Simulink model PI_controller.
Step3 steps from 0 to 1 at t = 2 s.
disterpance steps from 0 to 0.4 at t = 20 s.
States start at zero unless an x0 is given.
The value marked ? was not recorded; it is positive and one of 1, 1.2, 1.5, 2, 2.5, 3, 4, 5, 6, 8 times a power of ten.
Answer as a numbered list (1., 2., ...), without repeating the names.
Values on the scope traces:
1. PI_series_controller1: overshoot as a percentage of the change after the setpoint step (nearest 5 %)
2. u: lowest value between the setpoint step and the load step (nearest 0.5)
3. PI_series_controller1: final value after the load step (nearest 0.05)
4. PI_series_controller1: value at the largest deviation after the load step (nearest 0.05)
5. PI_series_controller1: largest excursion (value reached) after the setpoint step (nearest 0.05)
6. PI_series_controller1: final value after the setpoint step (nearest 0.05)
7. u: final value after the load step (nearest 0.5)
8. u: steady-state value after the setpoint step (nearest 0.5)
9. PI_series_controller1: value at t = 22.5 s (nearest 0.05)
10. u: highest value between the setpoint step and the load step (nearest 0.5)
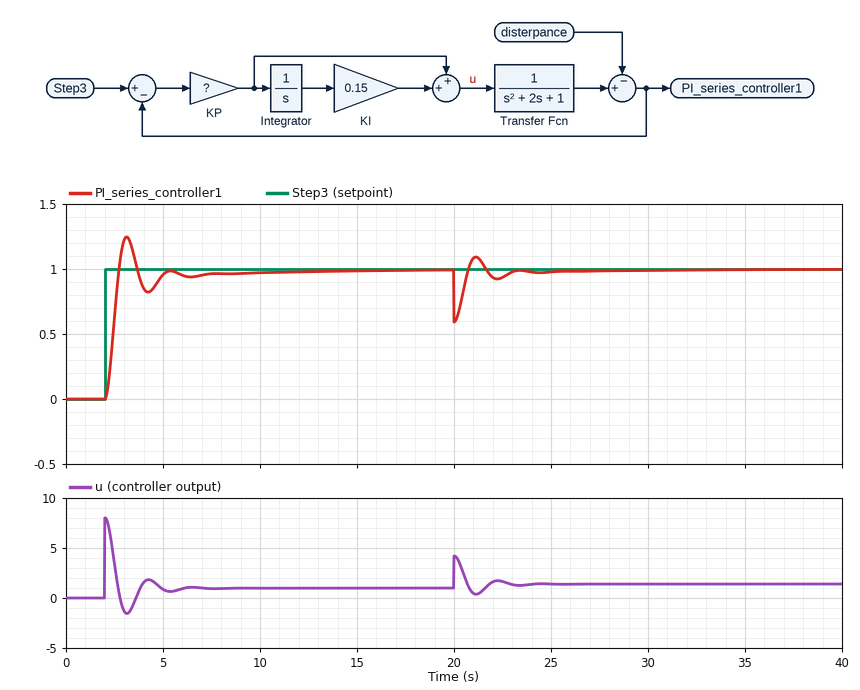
1. 25 %
2. -1.5
3. 1.00
4. 0.60
5. 1.25
6. 1.00
7. 1.5
8. 1.0
9. 0.95
10. 8.0
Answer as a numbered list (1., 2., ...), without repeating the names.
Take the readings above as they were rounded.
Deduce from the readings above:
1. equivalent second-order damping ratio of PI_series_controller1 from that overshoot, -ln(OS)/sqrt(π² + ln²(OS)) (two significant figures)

1. 0.40
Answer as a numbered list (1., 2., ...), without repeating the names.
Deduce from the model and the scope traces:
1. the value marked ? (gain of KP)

1. 8
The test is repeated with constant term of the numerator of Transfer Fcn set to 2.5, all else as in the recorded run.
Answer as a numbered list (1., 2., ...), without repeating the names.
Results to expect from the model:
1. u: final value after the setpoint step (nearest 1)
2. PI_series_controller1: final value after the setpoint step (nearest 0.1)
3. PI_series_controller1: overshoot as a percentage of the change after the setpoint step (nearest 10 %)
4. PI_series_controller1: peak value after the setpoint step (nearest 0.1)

1. 0
2. 1.0
3. 50 %
4. 1.5
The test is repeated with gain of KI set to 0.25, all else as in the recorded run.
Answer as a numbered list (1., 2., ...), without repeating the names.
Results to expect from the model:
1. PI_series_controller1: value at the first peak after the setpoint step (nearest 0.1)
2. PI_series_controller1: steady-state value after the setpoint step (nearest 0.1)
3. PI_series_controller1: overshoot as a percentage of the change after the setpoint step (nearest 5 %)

1. 1.3
2. 1.0
3. 30 %
